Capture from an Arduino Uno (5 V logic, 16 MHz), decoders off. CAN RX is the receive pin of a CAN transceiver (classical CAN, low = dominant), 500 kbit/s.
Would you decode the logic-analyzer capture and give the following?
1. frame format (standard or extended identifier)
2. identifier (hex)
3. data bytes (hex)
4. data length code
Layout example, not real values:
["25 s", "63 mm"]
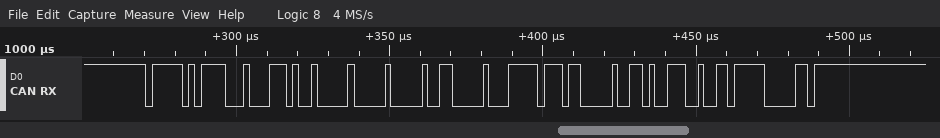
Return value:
["standard", "0x7EF", "E9 00 00 60 1F EC 06 9C", "8"]
